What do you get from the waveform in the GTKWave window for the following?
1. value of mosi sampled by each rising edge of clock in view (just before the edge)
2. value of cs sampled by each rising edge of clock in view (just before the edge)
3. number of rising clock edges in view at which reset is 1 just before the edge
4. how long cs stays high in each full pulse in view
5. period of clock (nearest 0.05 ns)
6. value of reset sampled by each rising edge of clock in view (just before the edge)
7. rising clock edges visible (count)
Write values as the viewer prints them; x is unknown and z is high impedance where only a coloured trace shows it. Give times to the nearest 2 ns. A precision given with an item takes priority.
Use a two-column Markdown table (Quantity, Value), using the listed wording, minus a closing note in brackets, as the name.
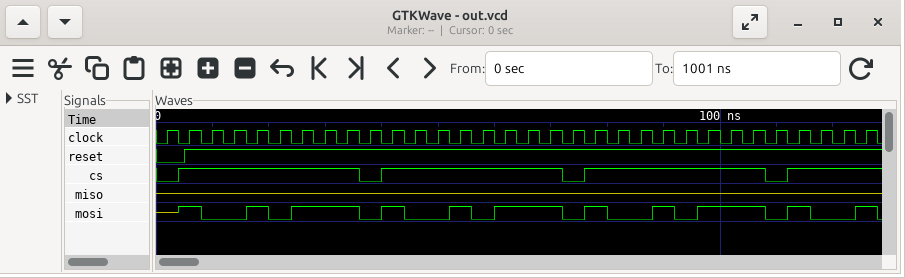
| Quantity | Value |
|---|---|
| value of mosi sampled by each rising edge of clock in view | z 1 0 0 1 0 1 1 1 0 1 0 0 1 0 1 1 1 0 1 0 0 1 0 1 1 1 0 1 0 0 1 |
| value of cs sampled by each rising edge of clock in view | 0 1 1 1 1 1 1 1 1 0 1 1 1 1 1 1 1 1 0 1 1 1 1 1 1 1 1 0 1 1 1 1 |
| number of rising clock edges in view at which reset is 1 just before the edge | 31 |
| how long cs stays high in each full pulse in view | 32 ns, 32 ns, 32 ns |
| period of clock | 4 ns |
| value of reset sampled by each rising edge of clock in view | 0 1 1 1 1 1 1 1 1 1 1 1 1 1 1 1 1 1 1 1 1 1 1 1 1 1 1 1 1 1 1 1 |
| rising clock edges visible | 32 |
